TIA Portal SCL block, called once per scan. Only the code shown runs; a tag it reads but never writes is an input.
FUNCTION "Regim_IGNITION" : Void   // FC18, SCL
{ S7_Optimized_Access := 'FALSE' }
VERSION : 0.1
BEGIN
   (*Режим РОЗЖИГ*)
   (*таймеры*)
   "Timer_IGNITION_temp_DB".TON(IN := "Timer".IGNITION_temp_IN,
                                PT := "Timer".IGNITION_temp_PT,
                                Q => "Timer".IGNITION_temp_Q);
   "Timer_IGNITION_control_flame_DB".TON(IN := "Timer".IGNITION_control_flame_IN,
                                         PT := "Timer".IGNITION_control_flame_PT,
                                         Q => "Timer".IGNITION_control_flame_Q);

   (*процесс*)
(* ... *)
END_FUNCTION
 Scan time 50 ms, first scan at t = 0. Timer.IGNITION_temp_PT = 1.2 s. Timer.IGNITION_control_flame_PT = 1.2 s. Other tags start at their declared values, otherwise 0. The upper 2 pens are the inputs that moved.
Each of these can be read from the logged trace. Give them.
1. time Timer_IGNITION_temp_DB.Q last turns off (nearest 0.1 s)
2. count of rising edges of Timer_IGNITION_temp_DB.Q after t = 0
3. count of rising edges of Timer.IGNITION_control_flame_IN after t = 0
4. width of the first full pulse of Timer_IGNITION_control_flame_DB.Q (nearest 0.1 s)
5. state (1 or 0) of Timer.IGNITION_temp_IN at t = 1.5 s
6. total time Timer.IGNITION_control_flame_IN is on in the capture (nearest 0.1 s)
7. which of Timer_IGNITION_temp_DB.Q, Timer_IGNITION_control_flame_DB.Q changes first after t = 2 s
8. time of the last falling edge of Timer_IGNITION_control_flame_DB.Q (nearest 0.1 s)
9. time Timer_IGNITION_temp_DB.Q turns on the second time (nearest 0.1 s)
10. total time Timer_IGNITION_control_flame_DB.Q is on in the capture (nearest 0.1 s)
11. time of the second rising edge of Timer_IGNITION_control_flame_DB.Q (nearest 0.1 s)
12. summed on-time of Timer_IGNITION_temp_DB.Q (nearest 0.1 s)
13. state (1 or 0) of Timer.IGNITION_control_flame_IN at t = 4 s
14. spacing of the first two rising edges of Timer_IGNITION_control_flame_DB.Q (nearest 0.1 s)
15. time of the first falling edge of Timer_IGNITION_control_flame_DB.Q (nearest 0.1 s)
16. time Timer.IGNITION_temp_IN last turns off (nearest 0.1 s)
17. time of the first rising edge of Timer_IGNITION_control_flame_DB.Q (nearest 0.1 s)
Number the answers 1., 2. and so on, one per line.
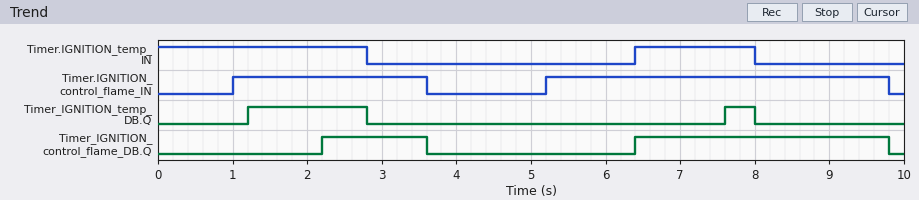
1. 8.0 s
2. 2
3. 2
4. 1.4 s
5. 1
6. 7.2 s
7. Timer_IGNITION_control_flame_DB.Q
8. 9.8 s
9. 7.6 s
10. 4.8 s
11. 6.4 s
12. 2.0 s
13. 0
14. 4.2 s
15. 3.6 s
16. 8.0 s
17. 2.2 s
